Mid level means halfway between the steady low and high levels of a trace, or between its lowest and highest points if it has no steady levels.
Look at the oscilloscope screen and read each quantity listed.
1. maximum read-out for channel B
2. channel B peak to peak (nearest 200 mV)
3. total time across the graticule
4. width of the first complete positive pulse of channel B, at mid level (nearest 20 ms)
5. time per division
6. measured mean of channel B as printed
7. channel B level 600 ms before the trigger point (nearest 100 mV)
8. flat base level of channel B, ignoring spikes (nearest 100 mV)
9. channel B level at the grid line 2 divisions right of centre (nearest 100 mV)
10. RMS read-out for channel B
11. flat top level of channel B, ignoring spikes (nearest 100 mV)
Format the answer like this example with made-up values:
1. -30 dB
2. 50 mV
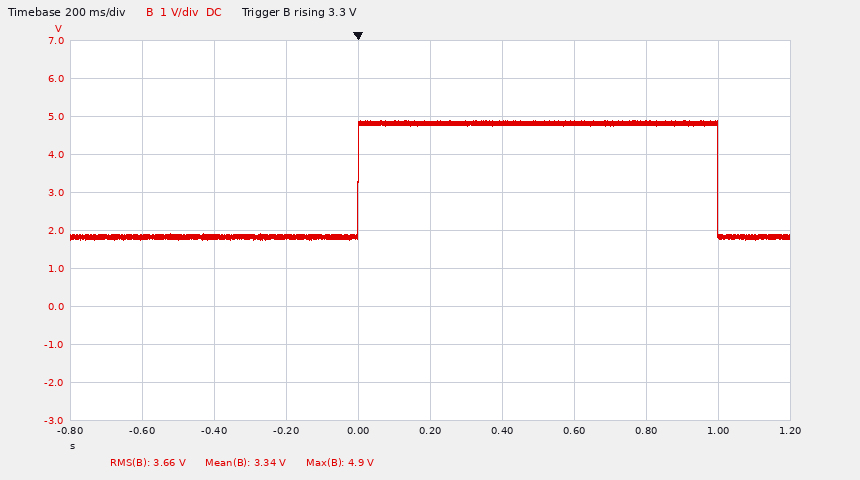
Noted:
1. 4.9 V
2. 3.2 V
3. 2 s
4. 1.00 s
5. 200 ms
6. 3.34 V
7. 1.8 V
8. 1.8 V
9. 4.8 V
10. 3.66 V
11. 4.8 V
